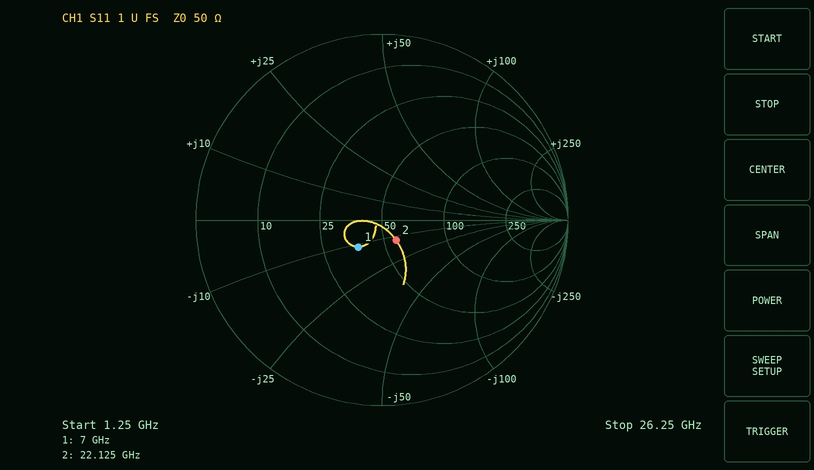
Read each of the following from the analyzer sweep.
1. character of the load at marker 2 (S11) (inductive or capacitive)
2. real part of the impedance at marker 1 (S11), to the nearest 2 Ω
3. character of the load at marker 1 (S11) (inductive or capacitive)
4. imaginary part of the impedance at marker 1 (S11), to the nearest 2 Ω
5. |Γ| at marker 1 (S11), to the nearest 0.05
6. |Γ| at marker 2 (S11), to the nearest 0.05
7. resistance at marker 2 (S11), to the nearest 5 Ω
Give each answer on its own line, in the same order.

capacitive
38 Ω
capacitive
-12 Ω
0.20
0.15
55 Ω
